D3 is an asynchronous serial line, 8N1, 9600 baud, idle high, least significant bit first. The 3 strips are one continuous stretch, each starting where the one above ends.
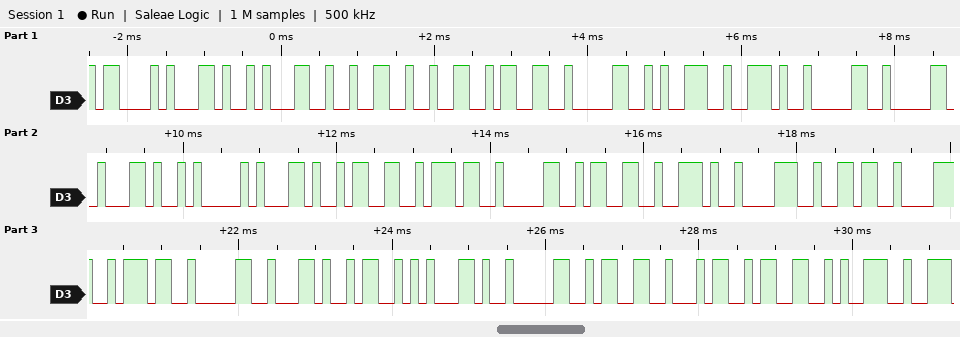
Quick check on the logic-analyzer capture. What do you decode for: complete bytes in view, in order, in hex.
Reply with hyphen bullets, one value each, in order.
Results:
- 43 2C 31 32 32 33 30 39 2E 30 30 2C 41 2C 33 37 30 33 2E 38 36 38 37 30 2C 53 2C 30 33 34 33 39
